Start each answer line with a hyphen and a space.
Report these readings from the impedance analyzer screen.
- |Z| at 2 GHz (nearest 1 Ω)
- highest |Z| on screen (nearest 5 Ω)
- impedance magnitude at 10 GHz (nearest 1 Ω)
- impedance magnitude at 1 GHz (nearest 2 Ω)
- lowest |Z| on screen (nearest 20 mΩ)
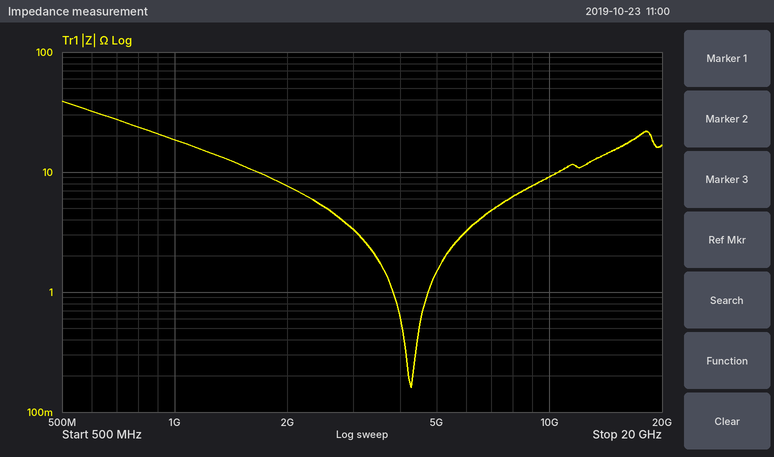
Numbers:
- 8 Ω
- 40 Ω
- 9 Ω
- 18 Ω
- 160 mΩ
